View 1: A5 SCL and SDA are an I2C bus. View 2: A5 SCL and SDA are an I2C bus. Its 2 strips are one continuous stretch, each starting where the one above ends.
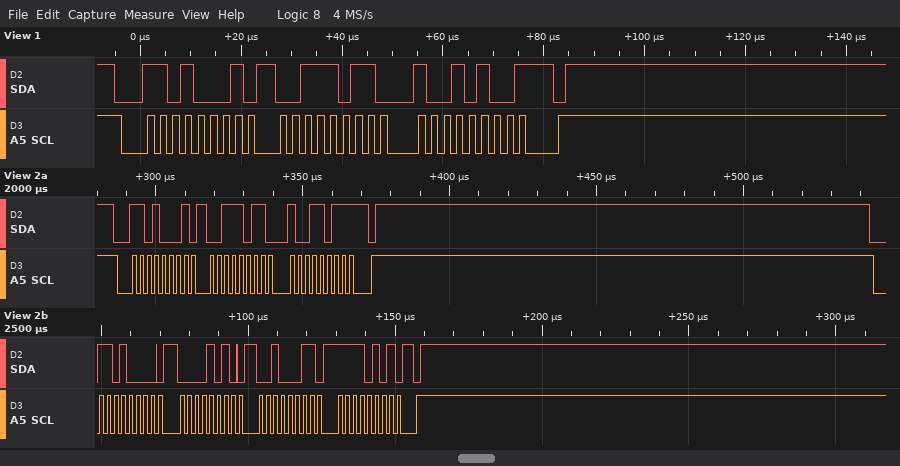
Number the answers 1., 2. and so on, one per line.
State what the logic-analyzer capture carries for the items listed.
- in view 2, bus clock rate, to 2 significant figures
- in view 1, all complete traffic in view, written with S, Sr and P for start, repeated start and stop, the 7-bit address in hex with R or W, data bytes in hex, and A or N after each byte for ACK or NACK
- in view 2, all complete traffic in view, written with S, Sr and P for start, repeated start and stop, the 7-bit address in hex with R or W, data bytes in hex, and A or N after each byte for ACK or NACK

1. 400 kHz
2. S 68R A 3B A 94 N P
3. S 68R A 3B A 9B N P S 68W A 0A A 23 A F5 A P
